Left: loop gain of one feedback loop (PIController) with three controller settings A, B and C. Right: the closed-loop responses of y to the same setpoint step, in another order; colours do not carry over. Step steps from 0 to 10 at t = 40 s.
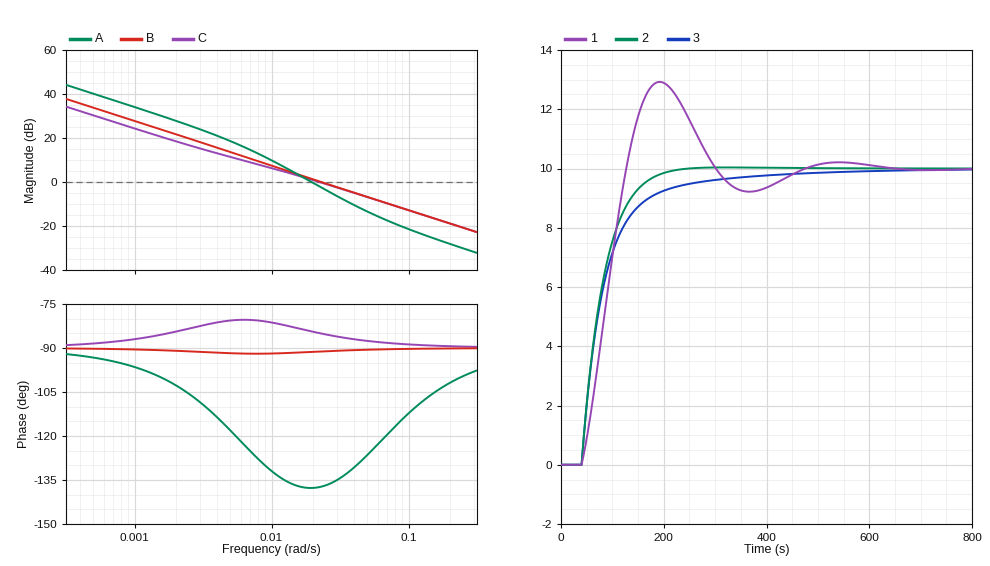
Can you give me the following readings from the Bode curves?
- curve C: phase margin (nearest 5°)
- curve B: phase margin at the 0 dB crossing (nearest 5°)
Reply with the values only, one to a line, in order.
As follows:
95°
90°
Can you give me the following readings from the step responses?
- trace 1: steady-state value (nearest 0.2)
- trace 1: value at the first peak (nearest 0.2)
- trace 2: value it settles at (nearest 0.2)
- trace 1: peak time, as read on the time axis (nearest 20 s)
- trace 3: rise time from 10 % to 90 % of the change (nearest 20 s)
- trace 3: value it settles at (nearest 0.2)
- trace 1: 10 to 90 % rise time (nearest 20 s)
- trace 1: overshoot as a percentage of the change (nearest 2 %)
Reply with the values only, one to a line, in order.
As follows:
10.0
13.0
10.0
200 s
120 s
10.0
60 s
30 %
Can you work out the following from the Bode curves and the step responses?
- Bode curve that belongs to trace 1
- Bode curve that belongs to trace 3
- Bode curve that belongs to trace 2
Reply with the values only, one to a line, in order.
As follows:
A
C
B
